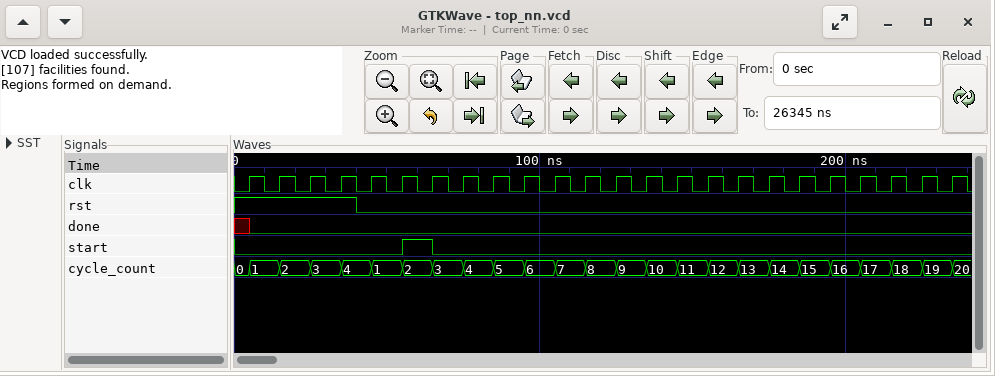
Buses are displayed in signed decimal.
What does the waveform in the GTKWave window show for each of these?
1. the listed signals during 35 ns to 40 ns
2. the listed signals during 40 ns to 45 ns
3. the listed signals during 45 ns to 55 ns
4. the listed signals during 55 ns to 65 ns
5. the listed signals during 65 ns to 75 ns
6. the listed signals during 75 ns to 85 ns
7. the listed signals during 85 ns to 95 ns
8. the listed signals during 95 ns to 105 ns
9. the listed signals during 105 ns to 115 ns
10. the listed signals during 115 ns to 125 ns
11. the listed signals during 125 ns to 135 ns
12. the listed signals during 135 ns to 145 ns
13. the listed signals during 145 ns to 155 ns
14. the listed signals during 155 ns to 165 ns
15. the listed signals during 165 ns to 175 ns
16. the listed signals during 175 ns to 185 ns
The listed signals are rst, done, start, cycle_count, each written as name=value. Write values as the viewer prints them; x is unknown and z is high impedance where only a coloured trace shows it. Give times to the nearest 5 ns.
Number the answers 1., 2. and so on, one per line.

1. rst=1, done=0, start=0, cycle_count=4
2. rst=0, done=0, start=0, cycle_count=4
3. rst=0, done=0, start=0, cycle_count=1
4. rst=0, done=0, start=1, cycle_count=2
5. rst=0, done=0, start=0, cycle_count=3
6. rst=0, done=0, start=0, cycle_count=4
7. rst=0, done=0, start=0, cycle_count=5
8. rst=0, done=0, start=0, cycle_count=6
9. rst=0, done=0, start=0, cycle_count=7
10. rst=0, done=0, start=0, cycle_count=8
11. rst=0, done=0, start=0, cycle_count=9
12. rst=0, done=0, start=0, cycle_count=10
13. rst=0, done=0, start=0, cycle_count=11
14. rst=0, done=0, start=0, cycle_count=12
15. rst=0, done=0, start=0, cycle_count=13
16. rst=0, done=0, start=0, cycle_count=14
